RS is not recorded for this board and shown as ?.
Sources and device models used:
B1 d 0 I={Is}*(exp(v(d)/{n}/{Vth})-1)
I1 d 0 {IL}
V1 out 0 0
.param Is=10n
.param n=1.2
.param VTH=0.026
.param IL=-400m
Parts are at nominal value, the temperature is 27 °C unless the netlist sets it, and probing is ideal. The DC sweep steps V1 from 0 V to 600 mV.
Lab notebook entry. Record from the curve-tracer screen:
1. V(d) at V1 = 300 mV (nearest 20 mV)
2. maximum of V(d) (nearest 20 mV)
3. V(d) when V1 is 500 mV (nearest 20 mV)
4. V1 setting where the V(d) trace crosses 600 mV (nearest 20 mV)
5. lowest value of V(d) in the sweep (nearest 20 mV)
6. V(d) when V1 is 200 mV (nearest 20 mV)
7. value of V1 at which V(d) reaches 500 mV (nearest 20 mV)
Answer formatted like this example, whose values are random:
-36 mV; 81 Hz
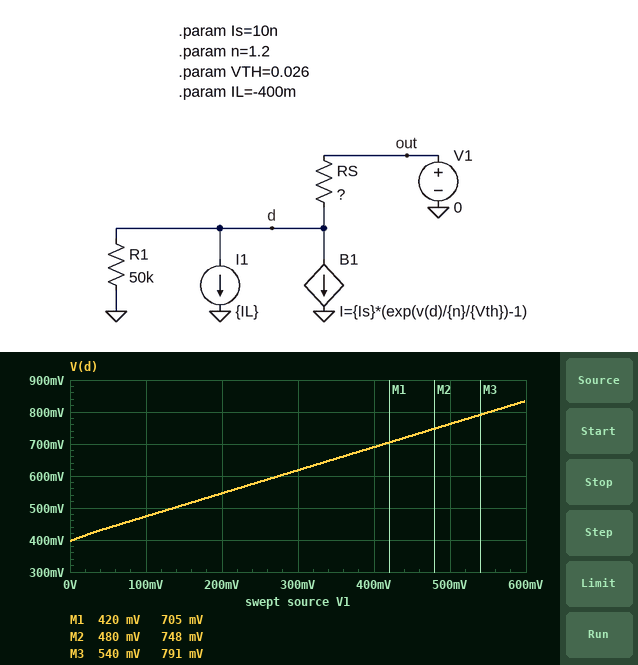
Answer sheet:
620 mV; 840 mV; 760 mV; 280 mV; 400 mV; 540 mV; 140 mV
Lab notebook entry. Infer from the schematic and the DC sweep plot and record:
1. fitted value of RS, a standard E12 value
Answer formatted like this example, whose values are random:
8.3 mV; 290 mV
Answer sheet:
1 Ω
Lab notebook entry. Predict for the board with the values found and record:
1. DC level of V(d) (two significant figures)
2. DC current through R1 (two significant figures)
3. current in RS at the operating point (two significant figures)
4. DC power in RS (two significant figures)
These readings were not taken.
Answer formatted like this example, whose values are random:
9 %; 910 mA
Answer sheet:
400 mV; 7.9 µA; 400 mA; 160 mW
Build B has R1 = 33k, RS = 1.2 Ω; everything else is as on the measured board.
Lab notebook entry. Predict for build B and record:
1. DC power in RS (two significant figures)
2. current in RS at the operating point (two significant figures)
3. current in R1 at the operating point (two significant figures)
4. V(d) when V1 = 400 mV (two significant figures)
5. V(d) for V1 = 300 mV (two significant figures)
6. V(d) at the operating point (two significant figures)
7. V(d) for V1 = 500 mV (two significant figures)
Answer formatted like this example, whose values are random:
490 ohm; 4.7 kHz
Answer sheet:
170 mW; 380 mA; 14 µA; 730 mV; 660 mV; 460 mV; 800 mV
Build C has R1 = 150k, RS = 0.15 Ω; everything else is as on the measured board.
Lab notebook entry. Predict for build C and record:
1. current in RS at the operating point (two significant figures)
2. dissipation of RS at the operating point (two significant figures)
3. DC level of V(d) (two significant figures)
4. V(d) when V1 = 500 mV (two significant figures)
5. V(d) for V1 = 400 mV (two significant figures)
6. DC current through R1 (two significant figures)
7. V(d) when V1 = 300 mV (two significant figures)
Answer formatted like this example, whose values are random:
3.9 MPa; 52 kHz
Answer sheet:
400 mA; 24 mW; 60 mV; 550 mV; 460 mV; 400 nA; 360 mV
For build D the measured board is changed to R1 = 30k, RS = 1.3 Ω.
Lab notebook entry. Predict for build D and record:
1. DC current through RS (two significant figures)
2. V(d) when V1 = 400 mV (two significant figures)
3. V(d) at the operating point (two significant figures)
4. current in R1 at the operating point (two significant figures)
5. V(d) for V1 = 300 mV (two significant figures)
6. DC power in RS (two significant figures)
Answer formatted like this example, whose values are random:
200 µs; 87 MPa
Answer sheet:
370 mA; 750 mV; 480 mV; 16 µA; 680 mV; 180 mW
